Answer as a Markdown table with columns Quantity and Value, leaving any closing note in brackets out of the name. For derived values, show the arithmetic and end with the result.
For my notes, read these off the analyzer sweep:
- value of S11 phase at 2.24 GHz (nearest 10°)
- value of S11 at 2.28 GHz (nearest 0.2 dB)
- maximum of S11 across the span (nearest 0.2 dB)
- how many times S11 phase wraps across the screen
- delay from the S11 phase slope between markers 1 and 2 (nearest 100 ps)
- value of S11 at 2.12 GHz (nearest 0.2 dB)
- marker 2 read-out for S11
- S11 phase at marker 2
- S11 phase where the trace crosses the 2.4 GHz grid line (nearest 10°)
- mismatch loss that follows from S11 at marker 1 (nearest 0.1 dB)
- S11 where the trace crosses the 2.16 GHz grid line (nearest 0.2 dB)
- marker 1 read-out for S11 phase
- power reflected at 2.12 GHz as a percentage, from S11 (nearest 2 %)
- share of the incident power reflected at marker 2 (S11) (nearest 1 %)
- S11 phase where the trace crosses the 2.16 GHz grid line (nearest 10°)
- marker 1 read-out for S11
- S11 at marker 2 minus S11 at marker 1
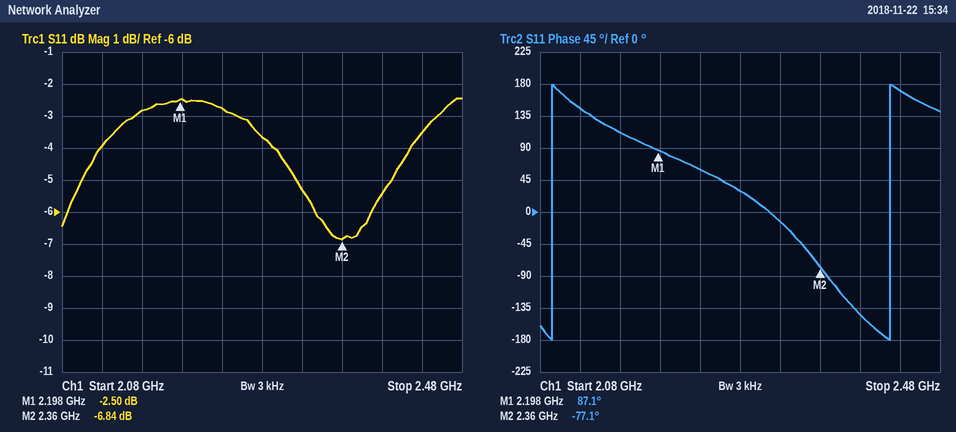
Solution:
| Quantity | Value |
|---|---|
| value of S11 phase at 2.24 GHz | 60° |
| value of S11 at 2.28 GHz | -3.6 dB |
| maximum of S11 across the span | -2.4 dB |
| how many times S11 phase wraps across the screen | 2 |
| delay from the S11 phase slope between markers 1 and 2 | −(-77.1° − (87.1°))/(360° × 162 MHz) ≈ 2.8 ns |
| value of S11 at 2.12 GHz | -4.0 dB |
| marker 2 read-out for S11 | -6.84 dB |
| S11 phase at marker 2 | -77.1° |
| S11 phase where the trace crosses the 2.4 GHz grid line | -140° |
| mismatch loss that follows from S11 at marker 1 | −10 log10(1 − 10^(-2.5/10)) ≈ 3.6 dB |
| S11 where the trace crosses the 2.16 GHz grid line | -2.8 dB |
| marker 1 read-out for S11 phase | 87.1° |
| power reflected at 2.12 GHz as a percentage, from S11 | 10^(-4/10) ≈ 40 % |
| share of the incident power reflected at marker 2 (S11) | 10^(-6.84/10) ≈ 21 % |
| S11 phase where the trace crosses the 2.16 GHz grid line | 110° |
| marker 1 read-out for S11 | -2.50 dB |
| S11 at marker 2 minus S11 at marker 1 | -6.84 − (-2.5) = -4.34 dB |
